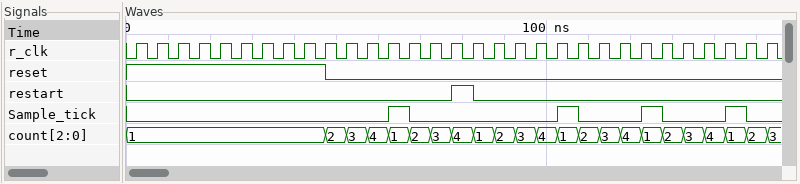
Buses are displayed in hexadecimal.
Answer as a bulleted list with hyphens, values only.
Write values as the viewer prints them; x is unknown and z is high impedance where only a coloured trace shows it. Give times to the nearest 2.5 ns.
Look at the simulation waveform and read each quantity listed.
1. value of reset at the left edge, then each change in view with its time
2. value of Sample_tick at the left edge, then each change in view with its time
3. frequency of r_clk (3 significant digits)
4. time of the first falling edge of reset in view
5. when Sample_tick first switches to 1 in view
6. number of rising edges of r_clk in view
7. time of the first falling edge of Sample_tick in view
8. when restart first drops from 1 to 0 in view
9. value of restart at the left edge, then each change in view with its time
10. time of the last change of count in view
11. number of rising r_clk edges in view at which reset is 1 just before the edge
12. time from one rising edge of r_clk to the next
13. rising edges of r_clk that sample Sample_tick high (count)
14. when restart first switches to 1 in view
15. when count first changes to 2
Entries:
- 1, 0 at 47.5 ns
- 0, 1 at 62.5 ns, 0 at 67.5 ns, 1 at 102.5 ns, 0 at 107.5 ns, 1 at 122.5 ns, 0 at 127.5 ns, 1 at 142.5 ns, 0 at 147.5 ns
- 200 MHz
- 47.5 ns
- 62.5 ns
- 31
- 67.5 ns
- 82.5 ns
- 0, 1 at 77.5 ns, 0 at 82.5 ns
- 152.5 ns
- 10
- 5 ns
- 4
- 77.5 ns
- 47.5 ns
